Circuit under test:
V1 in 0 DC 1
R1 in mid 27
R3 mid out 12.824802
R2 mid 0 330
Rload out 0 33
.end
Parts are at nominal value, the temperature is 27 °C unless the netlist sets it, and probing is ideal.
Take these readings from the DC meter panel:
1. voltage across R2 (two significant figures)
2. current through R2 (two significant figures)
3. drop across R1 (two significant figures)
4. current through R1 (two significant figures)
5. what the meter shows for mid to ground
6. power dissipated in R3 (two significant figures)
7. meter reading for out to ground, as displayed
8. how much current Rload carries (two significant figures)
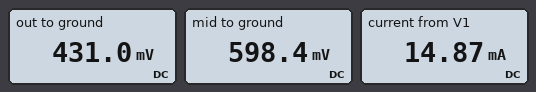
600 mV
1.8 mA
400 mV
15 mA
598.4 mV
2.2 mW
431.0 mV
13 mA
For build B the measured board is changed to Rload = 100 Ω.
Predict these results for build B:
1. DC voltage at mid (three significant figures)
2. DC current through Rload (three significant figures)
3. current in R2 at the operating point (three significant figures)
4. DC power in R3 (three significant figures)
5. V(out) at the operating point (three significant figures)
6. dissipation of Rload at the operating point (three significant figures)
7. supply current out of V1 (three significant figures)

757 mV
6.71 mA
2.29 mA
577 µW
671 mV
4.50 mW
9.00 mA
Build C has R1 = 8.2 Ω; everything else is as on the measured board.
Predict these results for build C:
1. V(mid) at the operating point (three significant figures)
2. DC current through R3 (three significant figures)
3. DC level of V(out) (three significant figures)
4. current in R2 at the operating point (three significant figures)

831 mV
18.1 mA
598 mV
2.52 mA
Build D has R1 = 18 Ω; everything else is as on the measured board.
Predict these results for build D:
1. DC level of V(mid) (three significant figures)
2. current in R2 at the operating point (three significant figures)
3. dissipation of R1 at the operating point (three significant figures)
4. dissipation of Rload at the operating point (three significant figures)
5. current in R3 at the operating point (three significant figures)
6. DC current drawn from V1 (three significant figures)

691 mV
2.09 mA
5.31 mW
7.50 mW
15.1 mA
17.2 mA
